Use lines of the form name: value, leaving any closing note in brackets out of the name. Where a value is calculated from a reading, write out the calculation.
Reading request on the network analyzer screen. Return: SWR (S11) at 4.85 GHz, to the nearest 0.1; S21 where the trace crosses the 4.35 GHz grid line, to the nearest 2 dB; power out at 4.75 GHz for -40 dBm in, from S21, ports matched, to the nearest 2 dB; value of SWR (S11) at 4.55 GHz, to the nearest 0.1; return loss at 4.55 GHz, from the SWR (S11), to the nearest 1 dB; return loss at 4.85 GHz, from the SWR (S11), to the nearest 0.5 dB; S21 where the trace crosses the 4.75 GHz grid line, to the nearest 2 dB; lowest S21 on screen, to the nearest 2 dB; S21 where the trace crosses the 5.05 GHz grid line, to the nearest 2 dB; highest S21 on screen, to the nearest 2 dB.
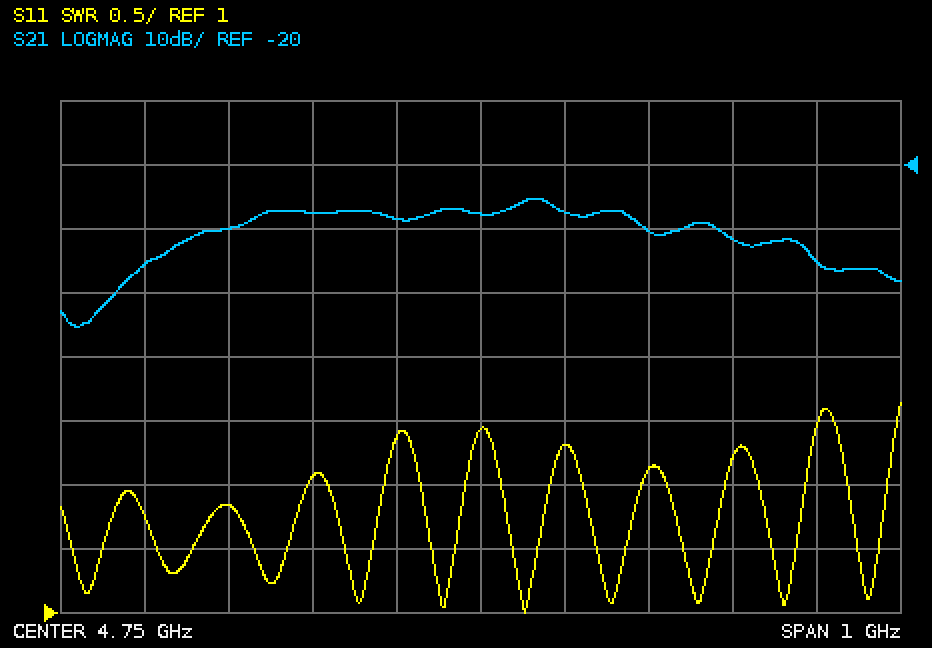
SWR (S11) at 4.85 GHz, to the nearest 0.1: 2.3
S21 where the trace crosses the 4.35 GHz grid line, to the nearest 2 dB: -36 dB
power out at 4.75 GHz for -40 dBm in, from S21, ports matched, to the nearest 2 dB: -40 dBm + (-28 dB) = -68 dBm
value of SWR (S11) at 4.55 GHz, to the nearest 0.1: 2.1
return loss at 4.55 GHz, from the SWR (S11), to the nearest 1 dB: −20 log10((2.1 − 1)/(2.1 + 1)) ≈ 9 dB
return loss at 4.85 GHz, from the SWR (S11), to the nearest 0.5 dB: −20 log10((2.3 − 1)/(2.3 + 1)) ≈ 8.09 dB, so 8.0 dB to the nearest 0.5 dB
S21 where the trace crosses the 4.75 GHz grid line, to the nearest 2 dB: -28 dB
lowest S21 on screen, to the nearest 2 dB: -46 dB
S21 where the trace crosses the 5.05 GHz grid line, to the nearest 2 dB: -32 dB
highest S21 on screen, to the nearest 2 dB: -26 dB
